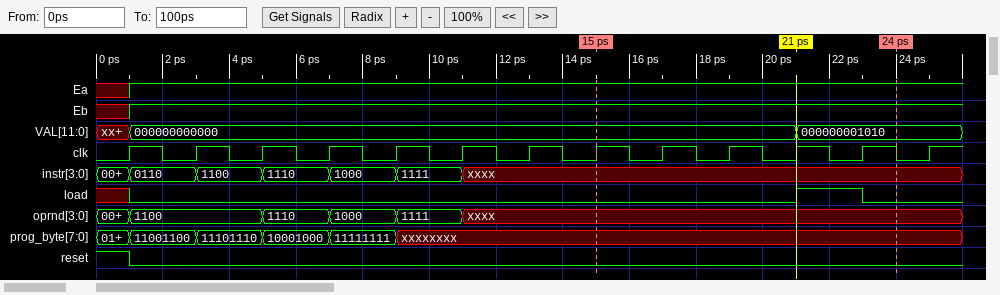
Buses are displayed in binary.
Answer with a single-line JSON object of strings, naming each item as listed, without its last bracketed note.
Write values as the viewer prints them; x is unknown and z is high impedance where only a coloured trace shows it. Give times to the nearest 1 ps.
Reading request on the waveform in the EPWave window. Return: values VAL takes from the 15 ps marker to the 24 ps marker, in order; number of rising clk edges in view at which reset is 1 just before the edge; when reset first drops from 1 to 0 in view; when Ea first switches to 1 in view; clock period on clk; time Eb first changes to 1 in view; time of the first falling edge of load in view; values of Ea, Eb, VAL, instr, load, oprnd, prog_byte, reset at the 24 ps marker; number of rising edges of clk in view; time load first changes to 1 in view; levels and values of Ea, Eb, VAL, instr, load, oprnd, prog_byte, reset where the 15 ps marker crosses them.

{"values VAL takes from the 15 ps marker to the 24 ps marker, in order": "000000000000, 000000001010", "number of rising clk edges in view at which reset is 1 just before the edge": "1", "when reset first drops from 1 to 0 in view": "1 ps", "when Ea first switches to 1 in view": "1 ps", "clock period on clk": "2 ps", "time Eb first changes to 1 in view": "1 ps", "time of the first falling edge of load in view": "23 ps", "values of Ea, Eb, VAL, instr, load, oprnd, prog_byte, reset at the 24 ps marker": "Ea=1, Eb=1, VAL=000000001010, instr=xxxx, load=0, oprnd=xxxx, prog_byte=xxxxxxxx, reset=0", "number of rising edges of clk in view": "13", "time load first changes to 1 in view": "21 ps", "levels and values of Ea, Eb, VAL, instr, load, oprnd, prog_byte, reset where the 15 ps marker crosses them": "Ea=1, Eb=1, VAL=000000000000, instr=xxxx, load=0, oprnd=xxxx, prog_byte=xxxxxxxx, reset=0"}
